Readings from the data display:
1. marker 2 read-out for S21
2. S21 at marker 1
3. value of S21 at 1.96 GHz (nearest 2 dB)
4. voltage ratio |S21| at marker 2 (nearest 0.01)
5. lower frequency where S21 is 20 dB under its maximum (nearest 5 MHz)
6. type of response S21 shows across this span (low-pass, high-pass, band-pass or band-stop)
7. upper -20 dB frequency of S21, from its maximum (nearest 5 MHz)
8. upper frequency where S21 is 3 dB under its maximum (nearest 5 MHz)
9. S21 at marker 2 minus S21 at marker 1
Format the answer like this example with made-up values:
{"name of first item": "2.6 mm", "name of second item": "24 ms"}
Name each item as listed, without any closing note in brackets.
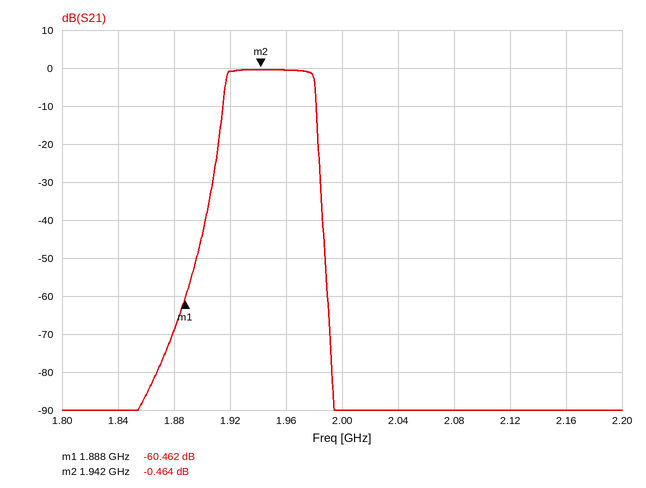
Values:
{"marker 2 read-out for S21": "-0.464 dB", "S21 at marker 1": "-60.462 dB", "value of S21 at 1.96 GHz": "0 dB", "voltage ratio |S21| at marker 2": "0.95", "lower frequency where S21 is 20 dB under its maximum": "1.910 GHz", "type of response S21 shows across this span": "band-pass", "upper -20 dB frequency of S21, from its maximum": "1.985 GHz", "upper frequency where S21 is 3 dB under its maximum": "1.980 GHz", "S21 at marker 2 minus S21 at marker 1": "59.998 dB"}
